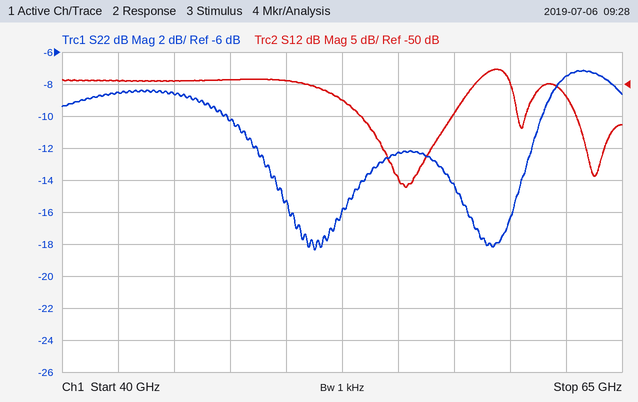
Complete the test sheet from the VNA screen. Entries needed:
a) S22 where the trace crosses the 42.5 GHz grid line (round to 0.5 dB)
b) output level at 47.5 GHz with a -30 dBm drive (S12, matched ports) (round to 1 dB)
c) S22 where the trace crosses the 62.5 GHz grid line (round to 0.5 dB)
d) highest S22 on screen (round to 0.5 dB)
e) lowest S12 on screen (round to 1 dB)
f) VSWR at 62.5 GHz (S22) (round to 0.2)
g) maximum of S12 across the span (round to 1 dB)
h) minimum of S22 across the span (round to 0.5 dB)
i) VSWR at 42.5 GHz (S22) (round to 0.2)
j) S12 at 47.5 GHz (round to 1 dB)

-8.5 dB
-79 dBm
-7.5 dB
-7.0 dB
-66 dB
2.4
-48 dB
-18.5 dB
2.2
-49 dB
